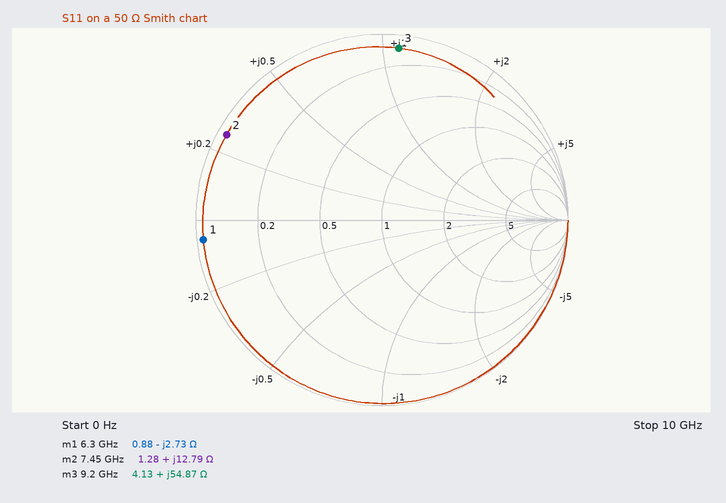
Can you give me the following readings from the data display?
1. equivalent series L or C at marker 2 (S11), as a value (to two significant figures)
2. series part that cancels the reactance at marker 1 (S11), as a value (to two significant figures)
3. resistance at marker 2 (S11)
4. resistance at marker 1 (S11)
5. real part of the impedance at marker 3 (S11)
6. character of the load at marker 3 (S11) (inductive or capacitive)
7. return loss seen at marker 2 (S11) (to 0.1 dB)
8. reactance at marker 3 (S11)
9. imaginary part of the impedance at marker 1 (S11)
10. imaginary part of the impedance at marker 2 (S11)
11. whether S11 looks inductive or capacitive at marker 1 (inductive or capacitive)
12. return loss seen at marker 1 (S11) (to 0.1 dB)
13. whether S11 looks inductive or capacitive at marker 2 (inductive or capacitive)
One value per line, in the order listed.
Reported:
270 pH
69 pH
1.28 Ω
0.88 Ω
4.13 Ω
inductive
0.4 dB
+54.87 Ω
-2.73 Ω
+12.79 Ω
capacitive
0.3 dB
inductive
